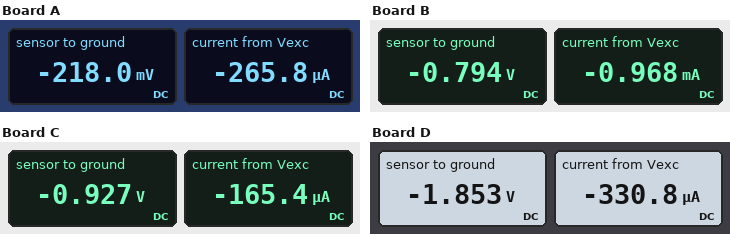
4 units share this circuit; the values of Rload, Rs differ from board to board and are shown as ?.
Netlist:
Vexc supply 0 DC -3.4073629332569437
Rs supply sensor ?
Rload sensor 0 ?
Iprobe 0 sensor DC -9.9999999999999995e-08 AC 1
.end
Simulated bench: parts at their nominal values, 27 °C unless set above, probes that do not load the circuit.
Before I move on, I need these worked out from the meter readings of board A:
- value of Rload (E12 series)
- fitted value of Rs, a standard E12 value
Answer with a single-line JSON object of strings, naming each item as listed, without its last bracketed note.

{"value of Rload": "820 Ω", "fitted value of Rs, a standard E12 value": "12 kΩ"}
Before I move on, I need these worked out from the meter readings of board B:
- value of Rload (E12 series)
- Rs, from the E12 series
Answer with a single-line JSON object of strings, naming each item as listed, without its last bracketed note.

{"value of Rload": "820 Ω", "Rs, from the E12 series": "2.7 kΩ"}
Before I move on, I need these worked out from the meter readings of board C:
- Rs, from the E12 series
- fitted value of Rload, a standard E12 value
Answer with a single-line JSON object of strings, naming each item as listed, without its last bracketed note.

{"Rs, from the E12 series": "15 kΩ", "fitted value of Rload, a standard E12 value": "5.6 kΩ"}
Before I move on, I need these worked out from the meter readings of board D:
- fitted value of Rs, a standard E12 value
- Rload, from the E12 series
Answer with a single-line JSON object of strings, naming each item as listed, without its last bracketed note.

{"fitted value of Rs, a standard E12 value": "4.7 kΩ", "Rload, from the E12 series": "5.6 kΩ"}
